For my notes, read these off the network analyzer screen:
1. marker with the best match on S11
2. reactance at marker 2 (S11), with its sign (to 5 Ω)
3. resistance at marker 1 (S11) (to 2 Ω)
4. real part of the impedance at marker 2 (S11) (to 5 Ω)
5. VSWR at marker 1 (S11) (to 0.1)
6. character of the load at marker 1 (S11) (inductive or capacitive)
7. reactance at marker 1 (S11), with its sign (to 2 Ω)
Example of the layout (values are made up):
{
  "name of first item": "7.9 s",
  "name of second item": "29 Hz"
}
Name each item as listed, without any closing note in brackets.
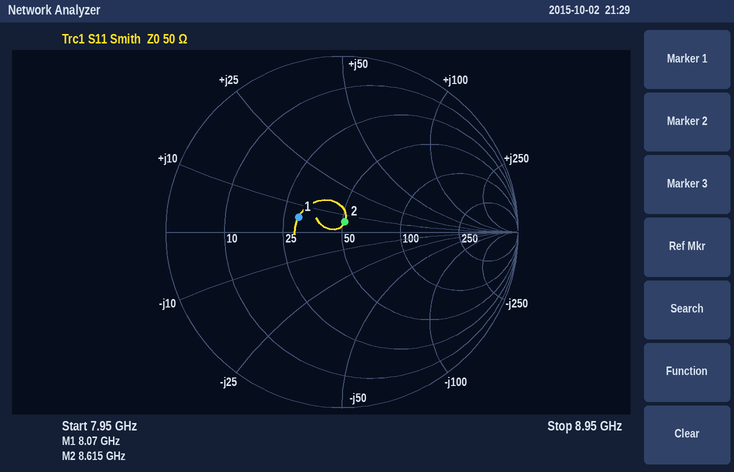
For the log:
{
  "marker with the best match on S11": "marker 2",
  "reactance at marker 2 (S11), with its sign": "+5 Ω",
  "resistance at marker 1 (S11)": "30 Ω",
  "real part of the impedance at marker 2 (S11)": "50 Ω",
  "VSWR at marker 1 (S11)": "1.7",
  "character of the load at marker 1 (S11)": "inductive",
  "reactance at marker 1 (S11), with its sign": "+6 Ω"
}
